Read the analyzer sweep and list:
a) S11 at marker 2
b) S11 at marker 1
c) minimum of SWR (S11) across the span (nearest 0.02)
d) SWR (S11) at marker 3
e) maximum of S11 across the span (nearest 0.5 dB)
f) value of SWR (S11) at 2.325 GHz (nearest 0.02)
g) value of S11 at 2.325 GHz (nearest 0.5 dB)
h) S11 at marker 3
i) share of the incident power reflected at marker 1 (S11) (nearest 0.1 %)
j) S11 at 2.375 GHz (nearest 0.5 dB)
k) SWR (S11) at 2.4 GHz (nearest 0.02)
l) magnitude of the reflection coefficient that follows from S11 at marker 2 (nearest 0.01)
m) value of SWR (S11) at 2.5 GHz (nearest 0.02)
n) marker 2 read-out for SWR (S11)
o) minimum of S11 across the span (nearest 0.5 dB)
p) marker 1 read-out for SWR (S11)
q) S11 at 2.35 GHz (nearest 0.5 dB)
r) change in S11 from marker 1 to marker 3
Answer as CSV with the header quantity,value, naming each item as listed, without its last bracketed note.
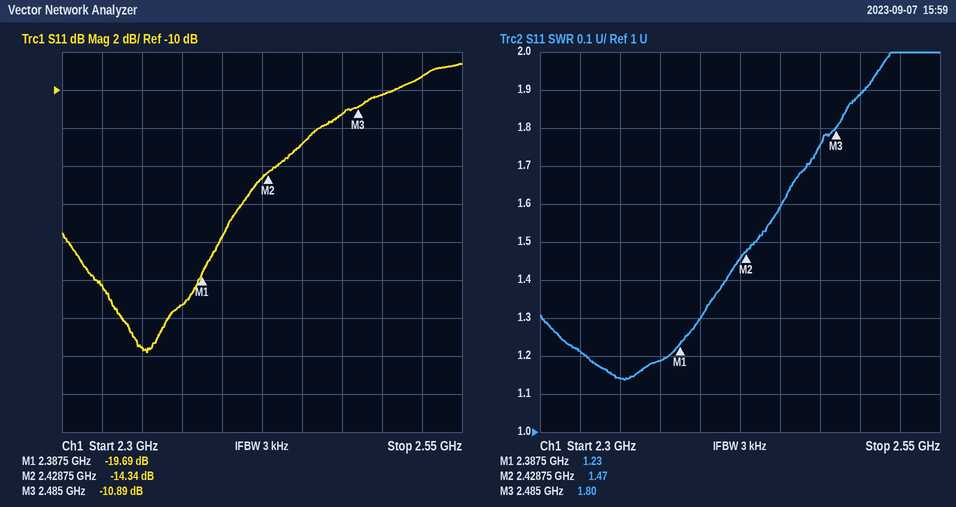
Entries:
quantity,value
S11 at marker 2,-14.34 dB
S11 at marker 1,-19.69 dB
minimum of SWR (S11) across the span,1.14
SWR (S11) at marker 3,1.80
maximum of S11 across the span,-8.5 dB
value of SWR (S11) at 2.325 GHz,1.22
value of S11 at 2.325 GHz,-20.5 dB
S11 at marker 3,-10.89 dB
share of the incident power reflected at marker 1 (S11),1.1 %
S11 at 2.375 GHz,-21.5 dB
SWR (S11) at 2.4 GHz,1.30
magnitude of the reflection coefficient that follows from S11 at marker 2,0.19
value of SWR (S11) at 2.5 GHz,1.88
marker 2 read-out for SWR,1.47
minimum of S11 across the span,-24.0 dB
marker 1 read-out for SWR,1.23
S11 at 2.35 GHz,-23.5 dB
change in S11 from marker 1 to marker 3,8.80 dB
